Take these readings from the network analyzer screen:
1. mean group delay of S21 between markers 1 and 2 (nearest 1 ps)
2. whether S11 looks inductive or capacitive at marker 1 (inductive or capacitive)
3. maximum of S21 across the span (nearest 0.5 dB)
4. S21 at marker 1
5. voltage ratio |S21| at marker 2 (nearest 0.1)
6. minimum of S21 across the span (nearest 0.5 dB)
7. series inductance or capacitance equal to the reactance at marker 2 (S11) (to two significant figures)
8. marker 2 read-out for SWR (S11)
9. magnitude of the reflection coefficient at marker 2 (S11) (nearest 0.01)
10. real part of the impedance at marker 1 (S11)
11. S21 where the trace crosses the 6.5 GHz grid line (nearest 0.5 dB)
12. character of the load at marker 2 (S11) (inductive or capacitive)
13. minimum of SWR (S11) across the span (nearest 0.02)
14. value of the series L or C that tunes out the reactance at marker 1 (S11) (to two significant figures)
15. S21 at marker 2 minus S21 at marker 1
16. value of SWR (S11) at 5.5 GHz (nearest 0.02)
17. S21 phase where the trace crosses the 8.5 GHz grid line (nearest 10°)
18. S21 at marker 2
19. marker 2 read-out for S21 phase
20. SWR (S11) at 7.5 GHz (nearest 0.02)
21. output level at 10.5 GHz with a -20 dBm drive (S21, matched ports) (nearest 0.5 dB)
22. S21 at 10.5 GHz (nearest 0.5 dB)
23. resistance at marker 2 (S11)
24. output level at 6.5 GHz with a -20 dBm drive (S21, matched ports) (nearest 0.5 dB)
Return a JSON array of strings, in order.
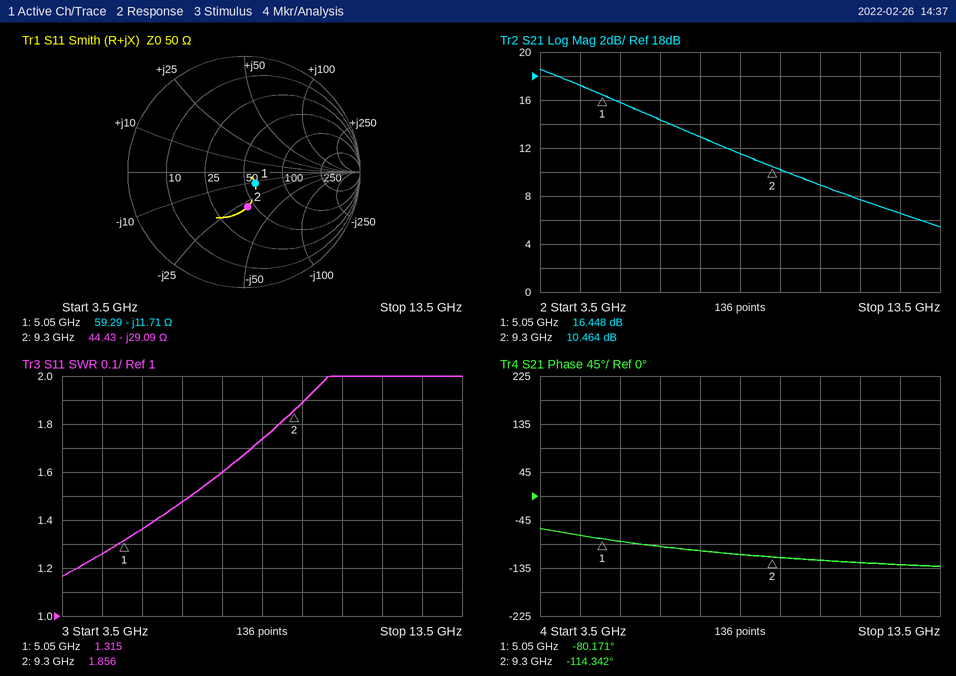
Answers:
["22 ps", "capacitive", "18.5 dB", "16.448 dB", "3.3", "5.5 dB", "590 fF", "1.856", "0.30", "59.29 Ω", "14.5 dB", "capacitive", "1.16", "370 pH", "-5.984 dB", "1.36", "-110°", "10.464 dB", "-114.342°", "1.60", "-11.0 dBm", "9.0 dB", "44.43 Ω", "-5.5 dBm"]
